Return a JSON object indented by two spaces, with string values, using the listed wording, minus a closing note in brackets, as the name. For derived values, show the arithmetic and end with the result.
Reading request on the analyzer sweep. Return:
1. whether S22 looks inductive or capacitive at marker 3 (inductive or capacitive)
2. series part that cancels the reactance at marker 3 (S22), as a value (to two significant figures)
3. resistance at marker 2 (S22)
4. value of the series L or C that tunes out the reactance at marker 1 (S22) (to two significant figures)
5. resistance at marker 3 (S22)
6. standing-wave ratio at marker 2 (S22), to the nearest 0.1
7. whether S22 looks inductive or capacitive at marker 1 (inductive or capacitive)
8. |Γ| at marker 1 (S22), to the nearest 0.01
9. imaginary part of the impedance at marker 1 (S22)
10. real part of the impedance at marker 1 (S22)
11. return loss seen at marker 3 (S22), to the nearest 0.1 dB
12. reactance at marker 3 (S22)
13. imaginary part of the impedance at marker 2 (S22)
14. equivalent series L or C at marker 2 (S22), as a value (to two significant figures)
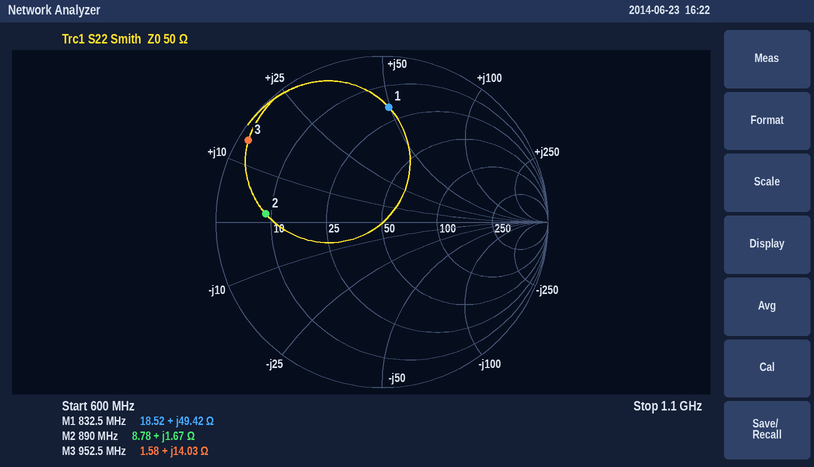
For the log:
{
  "whether S22 looks inductive or capacitive at marker 3": "inductive",
  "series part that cancels the reactance at marker 3 (S22), as a value": "C = 1/(2π × 952.5 MHz × 14.03 Ω) ≈ 12 pF",
  "resistance at marker 2": "8.78 Ω",
  "value of the series L or C that tunes out the reactance at marker 1 (S22)": "C = 1/(2π × 832.5 MHz × 49.42 Ω) ≈ 3.9 pF",
  "resistance at marker 3": "1.58 Ω",
  "standing-wave ratio at marker 2 (S22), to the nearest 0.1": "5.7",
  "whether S22 looks inductive or capacitive at marker 1": "inductive",
  "|Γ| at marker 1 (S22), to the nearest 0.01": "0.69",
  "imaginary part of the impedance at marker 1": "+49.42 Ω",
  "real part of the impedance at marker 1": "18.52 Ω",
  "return loss seen at marker 3 (S22), to the nearest 0.1 dB": "0.5 dB",
  "reactance at marker 3": "+14.03 Ω",
  "imaginary part of the impedance at marker 2": "+1.67 Ω",
  "equivalent series L or C at marker 2 (S22), as a value": "L = 1.67 Ω/(2π × 890 MHz) ≈ 299 pH, so 300 pH to two significant figures"
}
